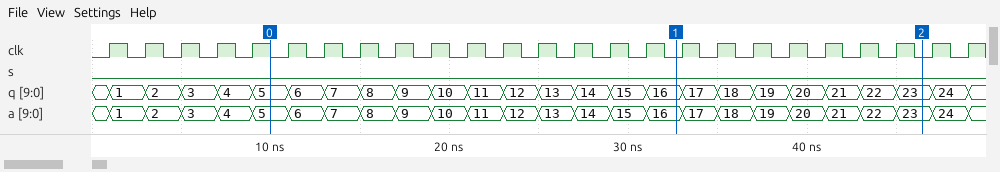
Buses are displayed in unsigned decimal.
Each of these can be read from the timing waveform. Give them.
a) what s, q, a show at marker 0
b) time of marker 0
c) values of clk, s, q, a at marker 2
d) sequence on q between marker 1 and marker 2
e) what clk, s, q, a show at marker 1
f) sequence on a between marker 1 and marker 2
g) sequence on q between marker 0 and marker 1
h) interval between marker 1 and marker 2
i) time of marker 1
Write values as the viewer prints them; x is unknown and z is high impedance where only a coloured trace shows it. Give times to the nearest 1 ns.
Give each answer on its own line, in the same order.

s=0, q=5, a=5
10 ns
clk=0, s=0, q=23, a=23
16, 17, 18, 19, 20, 21, 22, 23
clk=0, s=0, q=16, a=16
16, 17, 18, 19, 20, 21, 22, 23
5, 6, 7, 8, 9, 10, 11, 12, 13, 14, 15, 16
14 ns
33 ns
